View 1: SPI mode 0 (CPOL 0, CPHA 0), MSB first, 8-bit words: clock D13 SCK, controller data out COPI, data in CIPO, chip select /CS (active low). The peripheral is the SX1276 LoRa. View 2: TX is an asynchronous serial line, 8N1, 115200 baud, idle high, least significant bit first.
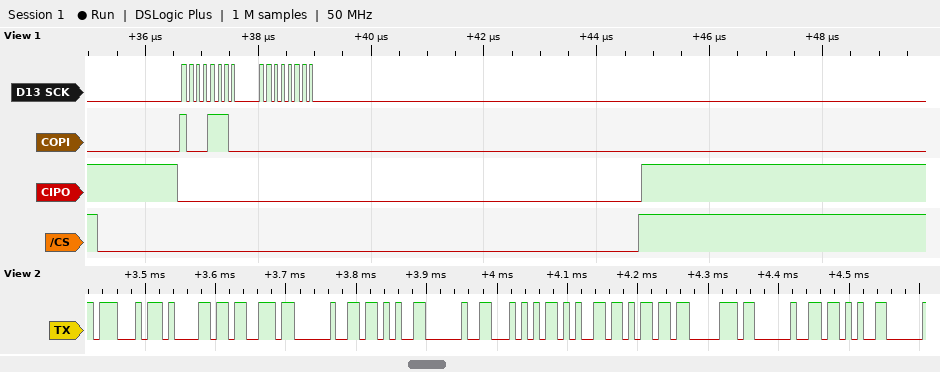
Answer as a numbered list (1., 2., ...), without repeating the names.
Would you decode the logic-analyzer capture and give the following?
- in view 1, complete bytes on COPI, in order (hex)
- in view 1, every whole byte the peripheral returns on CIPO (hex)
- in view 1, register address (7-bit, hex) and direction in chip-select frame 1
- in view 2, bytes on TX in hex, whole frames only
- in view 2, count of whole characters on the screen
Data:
1. 8E 00
2. 00 00
3. 0x0E write
4. 0x47 0x61 0x73 0x20 0x2B 0x20 0x54 0x65 0x6D 0x70 0x20 0x2B
5. 12
